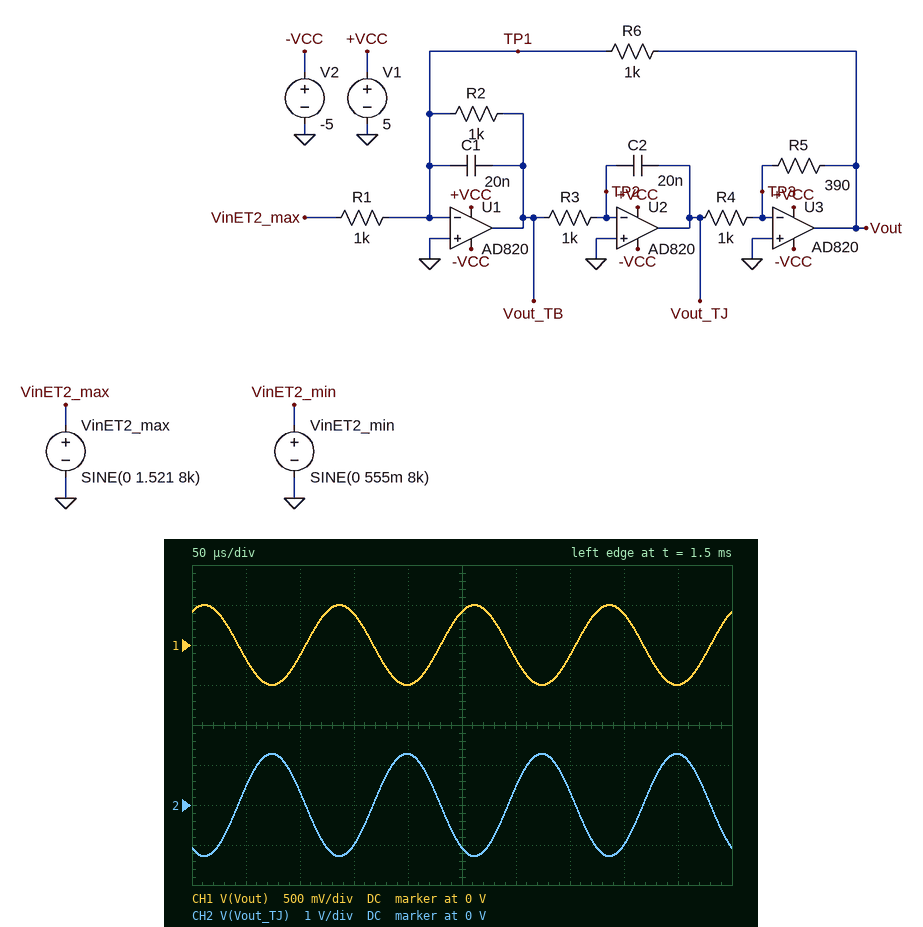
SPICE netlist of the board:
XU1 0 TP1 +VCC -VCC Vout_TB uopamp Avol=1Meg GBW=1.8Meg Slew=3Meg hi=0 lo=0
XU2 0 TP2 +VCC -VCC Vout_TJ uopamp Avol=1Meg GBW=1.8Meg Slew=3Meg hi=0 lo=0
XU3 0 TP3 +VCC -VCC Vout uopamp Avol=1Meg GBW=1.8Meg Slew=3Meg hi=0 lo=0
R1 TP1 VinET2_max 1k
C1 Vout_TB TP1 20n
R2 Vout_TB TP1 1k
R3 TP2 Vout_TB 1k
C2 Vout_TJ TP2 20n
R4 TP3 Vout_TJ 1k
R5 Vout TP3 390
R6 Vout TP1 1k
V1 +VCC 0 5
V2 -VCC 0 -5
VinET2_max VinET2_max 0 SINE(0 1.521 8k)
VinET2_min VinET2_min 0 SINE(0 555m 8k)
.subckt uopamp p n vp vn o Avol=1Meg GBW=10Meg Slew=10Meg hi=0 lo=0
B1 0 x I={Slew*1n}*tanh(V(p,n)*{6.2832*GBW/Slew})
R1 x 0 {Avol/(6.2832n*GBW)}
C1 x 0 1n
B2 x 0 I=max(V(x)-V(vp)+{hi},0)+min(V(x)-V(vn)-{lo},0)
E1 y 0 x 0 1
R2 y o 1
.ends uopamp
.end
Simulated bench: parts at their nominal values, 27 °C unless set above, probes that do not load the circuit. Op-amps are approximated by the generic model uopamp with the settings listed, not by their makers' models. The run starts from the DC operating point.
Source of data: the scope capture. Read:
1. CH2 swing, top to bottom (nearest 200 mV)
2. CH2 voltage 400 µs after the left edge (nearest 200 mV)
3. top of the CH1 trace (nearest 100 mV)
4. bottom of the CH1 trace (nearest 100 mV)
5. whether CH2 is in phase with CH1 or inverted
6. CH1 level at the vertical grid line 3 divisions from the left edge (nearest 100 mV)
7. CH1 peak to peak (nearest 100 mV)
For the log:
2.6 V
-1.0 V
500 mV
-500 mV
inverted
400 mV
1.0 V
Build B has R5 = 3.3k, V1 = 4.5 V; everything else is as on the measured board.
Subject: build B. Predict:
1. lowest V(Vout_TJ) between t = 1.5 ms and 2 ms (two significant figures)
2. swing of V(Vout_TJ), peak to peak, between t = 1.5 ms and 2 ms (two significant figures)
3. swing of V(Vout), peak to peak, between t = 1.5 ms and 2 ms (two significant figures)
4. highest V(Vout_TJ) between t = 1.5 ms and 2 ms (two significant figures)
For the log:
-620 mV
1.2 V
4.1 V
620 mV
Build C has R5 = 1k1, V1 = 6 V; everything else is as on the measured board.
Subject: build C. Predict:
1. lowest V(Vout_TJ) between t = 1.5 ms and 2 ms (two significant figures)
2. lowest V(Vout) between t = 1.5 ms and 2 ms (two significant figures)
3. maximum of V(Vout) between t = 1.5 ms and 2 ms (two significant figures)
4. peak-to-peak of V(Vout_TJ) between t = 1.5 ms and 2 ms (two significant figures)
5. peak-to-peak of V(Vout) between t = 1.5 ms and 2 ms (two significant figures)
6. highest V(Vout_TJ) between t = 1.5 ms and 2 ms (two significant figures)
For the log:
-1.5 V
-1.7 V
1.7 V
3.1 V
3.4 V
1.5 V
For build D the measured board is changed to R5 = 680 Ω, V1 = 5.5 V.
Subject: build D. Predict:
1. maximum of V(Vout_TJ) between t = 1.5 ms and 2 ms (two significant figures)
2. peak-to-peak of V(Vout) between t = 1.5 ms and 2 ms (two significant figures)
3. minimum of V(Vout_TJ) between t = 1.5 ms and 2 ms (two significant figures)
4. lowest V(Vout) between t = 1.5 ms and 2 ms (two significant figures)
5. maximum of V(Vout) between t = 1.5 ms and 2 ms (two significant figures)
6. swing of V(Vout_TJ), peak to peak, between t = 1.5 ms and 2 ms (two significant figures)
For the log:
1.4 V
2.0 V
-1.4 V
-980 mV
980 mV
2.9 V
